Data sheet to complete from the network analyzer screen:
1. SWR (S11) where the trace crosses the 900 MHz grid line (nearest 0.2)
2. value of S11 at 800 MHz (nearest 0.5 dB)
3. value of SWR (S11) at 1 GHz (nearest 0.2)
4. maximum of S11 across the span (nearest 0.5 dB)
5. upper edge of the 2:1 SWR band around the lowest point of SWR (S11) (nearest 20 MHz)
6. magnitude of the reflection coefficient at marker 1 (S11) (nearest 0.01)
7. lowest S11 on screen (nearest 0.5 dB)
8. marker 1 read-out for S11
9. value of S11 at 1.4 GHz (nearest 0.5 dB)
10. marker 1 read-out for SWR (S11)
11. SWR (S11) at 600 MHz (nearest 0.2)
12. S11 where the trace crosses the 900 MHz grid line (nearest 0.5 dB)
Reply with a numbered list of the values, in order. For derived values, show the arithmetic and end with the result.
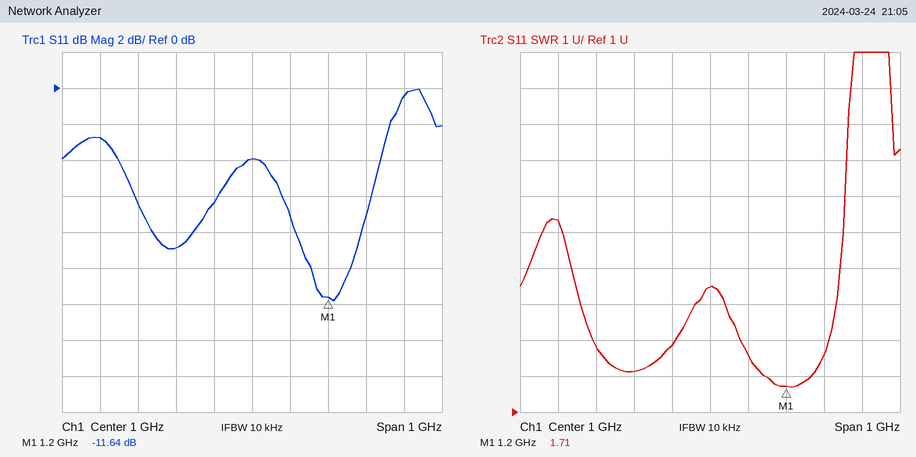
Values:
1. 2.8
2. -9.0 dB
3. 4.4
4. 0.0 dB
5. 1.26 GHz
6. 10^(-11.64/20) ≈ 0.26
7. -12.0 dB
8. -11.64 dB
9. -0.5 dB
10. 1.71
11. 6.4
12. -6.5 dB
